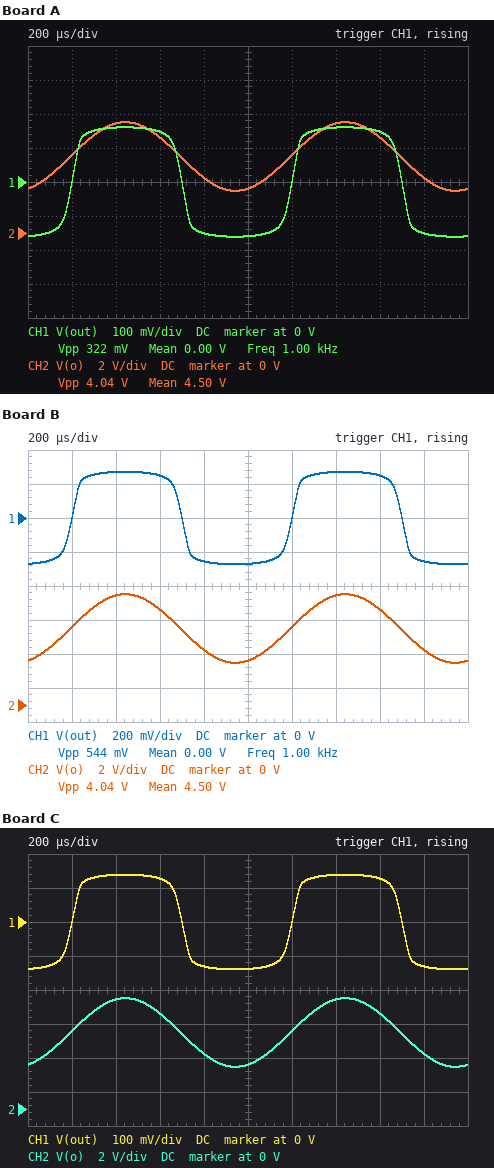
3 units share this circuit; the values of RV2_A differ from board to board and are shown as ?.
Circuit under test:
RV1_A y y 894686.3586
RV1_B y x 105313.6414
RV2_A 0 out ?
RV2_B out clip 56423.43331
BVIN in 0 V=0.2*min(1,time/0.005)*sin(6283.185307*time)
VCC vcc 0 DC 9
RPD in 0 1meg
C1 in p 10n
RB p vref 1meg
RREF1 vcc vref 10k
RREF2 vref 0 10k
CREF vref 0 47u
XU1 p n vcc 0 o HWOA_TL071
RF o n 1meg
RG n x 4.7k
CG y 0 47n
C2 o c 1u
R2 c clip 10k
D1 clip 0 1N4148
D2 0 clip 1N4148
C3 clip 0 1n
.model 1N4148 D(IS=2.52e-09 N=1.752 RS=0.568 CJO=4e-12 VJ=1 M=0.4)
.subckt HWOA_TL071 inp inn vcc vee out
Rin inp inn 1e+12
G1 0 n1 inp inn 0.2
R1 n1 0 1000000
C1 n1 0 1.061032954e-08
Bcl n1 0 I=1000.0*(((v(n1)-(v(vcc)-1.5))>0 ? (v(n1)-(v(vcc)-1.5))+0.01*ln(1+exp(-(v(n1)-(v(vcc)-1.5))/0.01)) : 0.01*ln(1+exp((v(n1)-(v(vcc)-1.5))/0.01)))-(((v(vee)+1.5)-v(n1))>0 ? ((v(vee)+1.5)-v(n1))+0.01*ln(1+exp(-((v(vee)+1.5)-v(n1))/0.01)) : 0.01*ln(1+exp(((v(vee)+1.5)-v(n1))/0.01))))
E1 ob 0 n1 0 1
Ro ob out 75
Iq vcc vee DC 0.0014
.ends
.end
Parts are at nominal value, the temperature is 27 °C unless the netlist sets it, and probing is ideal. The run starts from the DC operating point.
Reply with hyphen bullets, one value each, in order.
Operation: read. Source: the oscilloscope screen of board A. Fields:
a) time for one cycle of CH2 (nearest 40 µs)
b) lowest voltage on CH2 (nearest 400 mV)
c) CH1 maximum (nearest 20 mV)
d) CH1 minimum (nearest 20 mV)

- 1.00 ms
- 2.4 V
- 160 mV
- -160 mV
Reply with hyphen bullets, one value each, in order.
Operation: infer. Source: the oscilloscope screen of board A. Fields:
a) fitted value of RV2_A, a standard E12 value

- 27 kΩ
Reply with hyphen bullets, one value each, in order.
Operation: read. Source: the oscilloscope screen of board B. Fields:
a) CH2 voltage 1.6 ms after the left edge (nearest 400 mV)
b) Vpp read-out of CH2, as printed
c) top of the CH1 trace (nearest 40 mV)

- 5.6 V
- 4.04 V
- 280 mV
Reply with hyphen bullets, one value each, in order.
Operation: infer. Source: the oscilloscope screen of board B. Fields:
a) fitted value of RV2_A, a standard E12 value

- 68 kΩ
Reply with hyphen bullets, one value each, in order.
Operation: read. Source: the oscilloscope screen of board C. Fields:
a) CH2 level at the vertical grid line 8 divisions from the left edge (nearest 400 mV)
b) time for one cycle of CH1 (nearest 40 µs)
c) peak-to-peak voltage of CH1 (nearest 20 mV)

- 5.6 V
- 1.00 ms
- 280 mV
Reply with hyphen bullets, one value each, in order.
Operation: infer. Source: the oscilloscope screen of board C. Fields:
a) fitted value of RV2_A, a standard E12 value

- 22 kΩ
